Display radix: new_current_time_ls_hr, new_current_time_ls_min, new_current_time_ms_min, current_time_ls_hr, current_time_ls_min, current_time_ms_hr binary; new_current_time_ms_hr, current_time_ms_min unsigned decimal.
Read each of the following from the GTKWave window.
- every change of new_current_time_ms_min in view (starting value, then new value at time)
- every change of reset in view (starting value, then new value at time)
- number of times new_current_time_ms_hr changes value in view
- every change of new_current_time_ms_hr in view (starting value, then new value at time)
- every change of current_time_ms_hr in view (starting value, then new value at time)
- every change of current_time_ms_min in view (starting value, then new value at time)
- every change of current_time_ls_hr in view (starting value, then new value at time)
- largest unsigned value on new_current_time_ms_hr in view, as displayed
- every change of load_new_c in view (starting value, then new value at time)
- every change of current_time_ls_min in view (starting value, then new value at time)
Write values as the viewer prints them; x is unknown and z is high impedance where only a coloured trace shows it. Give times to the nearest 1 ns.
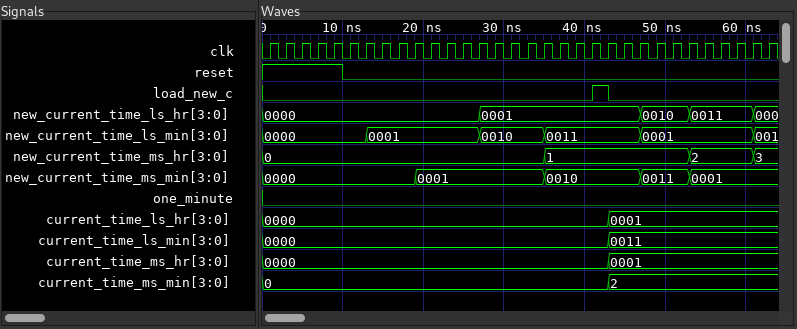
0000, 0001 at 19 ns, 0010 at 35 ns, 0011 at 47 ns, 0001 at 53 ns
1, 0 at 10 ns
3
0, 1 at 35 ns, 2 at 53 ns, 3 at 61 ns
0000, 0001 at 43 ns
0, 2 at 43 ns
0000, 0001 at 43 ns
3
0, 1 at 41 ns, 0 at 43 ns
0000, 0011 at 43 ns
